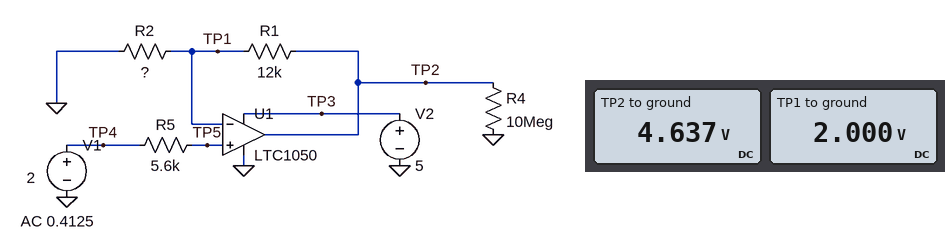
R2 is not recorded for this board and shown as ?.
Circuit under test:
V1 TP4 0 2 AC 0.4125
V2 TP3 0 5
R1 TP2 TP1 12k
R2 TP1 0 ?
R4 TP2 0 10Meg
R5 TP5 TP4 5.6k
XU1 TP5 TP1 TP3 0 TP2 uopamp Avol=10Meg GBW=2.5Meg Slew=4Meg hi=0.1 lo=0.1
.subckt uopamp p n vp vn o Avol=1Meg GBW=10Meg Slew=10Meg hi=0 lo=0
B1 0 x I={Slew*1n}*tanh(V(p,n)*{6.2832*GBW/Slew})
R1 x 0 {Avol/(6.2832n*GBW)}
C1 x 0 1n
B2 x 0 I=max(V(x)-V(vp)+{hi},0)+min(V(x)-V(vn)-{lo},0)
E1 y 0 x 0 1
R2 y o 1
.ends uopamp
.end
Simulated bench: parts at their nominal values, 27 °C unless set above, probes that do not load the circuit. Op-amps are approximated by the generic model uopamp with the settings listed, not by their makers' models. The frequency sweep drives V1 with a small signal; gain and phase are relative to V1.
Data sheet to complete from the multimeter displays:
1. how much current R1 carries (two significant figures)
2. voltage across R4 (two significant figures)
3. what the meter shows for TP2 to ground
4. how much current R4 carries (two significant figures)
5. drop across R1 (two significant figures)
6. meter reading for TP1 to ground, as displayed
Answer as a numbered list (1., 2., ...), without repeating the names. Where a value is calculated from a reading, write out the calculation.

1. (4.637 V - 2 V) / 12 kΩ = 220 µA
2. 4.637 V = 4.6 V
3. 4.637 V
4. (4.637 V) / 10 MΩ = 460 nA
5. 4.637 V - 2 V = 2.6 V
6. 2.000 V
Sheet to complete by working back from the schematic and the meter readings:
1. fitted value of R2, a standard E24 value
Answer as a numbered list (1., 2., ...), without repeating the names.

1. 9.1 kΩ
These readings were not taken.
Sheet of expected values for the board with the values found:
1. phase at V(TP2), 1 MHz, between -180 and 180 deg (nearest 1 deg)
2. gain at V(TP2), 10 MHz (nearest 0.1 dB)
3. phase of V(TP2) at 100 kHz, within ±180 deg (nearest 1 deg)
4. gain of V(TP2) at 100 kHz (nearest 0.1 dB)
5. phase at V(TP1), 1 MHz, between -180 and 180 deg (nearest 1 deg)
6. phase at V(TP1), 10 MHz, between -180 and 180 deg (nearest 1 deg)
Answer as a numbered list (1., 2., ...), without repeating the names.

1. -43 deg
2. -12.1 dB
3. -5 deg
4. 7.3 dB
5. -43 deg
6. -84 deg
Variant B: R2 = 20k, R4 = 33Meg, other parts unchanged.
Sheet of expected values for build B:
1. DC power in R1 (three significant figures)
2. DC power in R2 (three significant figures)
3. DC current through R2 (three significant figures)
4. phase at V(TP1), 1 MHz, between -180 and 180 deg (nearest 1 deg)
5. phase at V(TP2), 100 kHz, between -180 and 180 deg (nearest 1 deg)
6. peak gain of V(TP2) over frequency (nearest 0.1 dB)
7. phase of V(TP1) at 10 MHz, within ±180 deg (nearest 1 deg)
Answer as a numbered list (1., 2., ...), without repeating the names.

1. 120 µW
2. 200 µW
3. 100 µA
4. -33 deg
5. -4 deg
6. 4.1 dB
7. -81 deg
